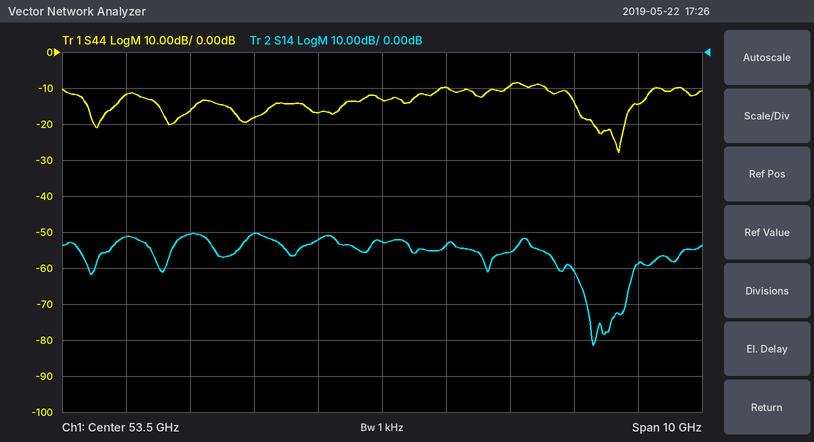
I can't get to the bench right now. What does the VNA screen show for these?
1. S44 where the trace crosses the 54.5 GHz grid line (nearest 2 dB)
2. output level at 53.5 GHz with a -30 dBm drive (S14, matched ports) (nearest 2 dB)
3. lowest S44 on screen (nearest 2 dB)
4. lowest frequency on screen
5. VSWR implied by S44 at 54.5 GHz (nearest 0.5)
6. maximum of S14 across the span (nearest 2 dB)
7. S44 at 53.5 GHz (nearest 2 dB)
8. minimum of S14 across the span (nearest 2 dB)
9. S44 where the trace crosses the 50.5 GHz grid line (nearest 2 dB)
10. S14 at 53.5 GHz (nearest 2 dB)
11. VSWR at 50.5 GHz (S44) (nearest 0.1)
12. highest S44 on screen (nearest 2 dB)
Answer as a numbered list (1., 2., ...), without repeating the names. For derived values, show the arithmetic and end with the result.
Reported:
1. -10 dB
2. -30 dBm + (-52 dB) = -82 dBm
3. -28 dB
4. 48.5 GHz
5. |Γ| = 10^(-10/20) = 0.3162; VSWR = (1 + 0.3162)/(1 − 0.3162) ≈ 1.92, so 2.0 to the nearest 0.5
6. -50 dB
7. -14 dB
8. -82 dB
9. -16 dB
10. -52 dB
11. |Γ| = 10^(-16/20) = 0.1585; VSWR = (1 + 0.1585)/(1 − 0.1585) ≈ 1.4
12. -8 dB
